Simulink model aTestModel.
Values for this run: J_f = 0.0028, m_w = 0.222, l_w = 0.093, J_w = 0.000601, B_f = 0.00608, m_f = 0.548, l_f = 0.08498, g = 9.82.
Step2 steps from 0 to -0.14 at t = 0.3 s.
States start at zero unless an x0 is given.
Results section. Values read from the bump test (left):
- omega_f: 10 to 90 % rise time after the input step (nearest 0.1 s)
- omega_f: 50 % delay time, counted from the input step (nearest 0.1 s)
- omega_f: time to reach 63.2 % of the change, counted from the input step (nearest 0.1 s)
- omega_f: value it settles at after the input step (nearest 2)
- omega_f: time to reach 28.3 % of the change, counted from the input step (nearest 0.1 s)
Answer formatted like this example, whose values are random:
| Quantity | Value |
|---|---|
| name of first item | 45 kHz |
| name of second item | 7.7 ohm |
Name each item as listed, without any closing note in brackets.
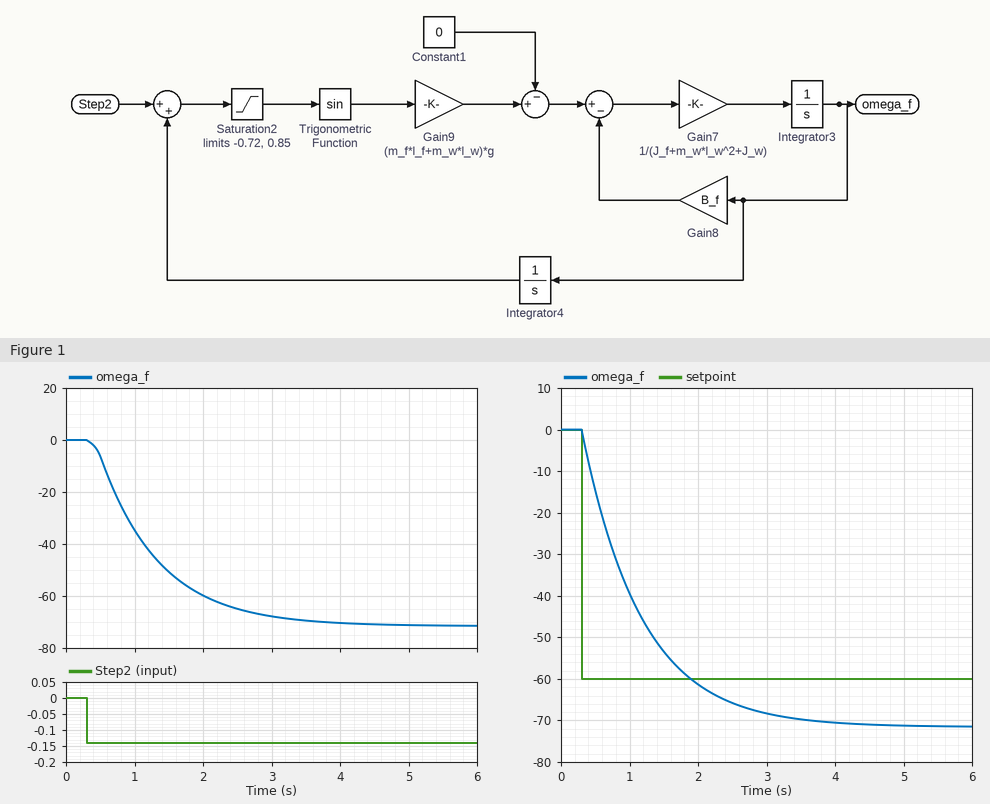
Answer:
| Quantity | Value |
|---|---|
| omega_f: 10 to 90 % rise time after the input step | 1.9 s |
| omega_f: 50 % delay time, counted from the input step | 0.7 s |
| omega_f: time to reach 63.2 % of the change, counted from the input step | 1.0 s |
| omega_f: value it settles at after the input step | -72 |
| omega_f: time to reach 28.3 % of the change, counted from the input step | 0.4 s |
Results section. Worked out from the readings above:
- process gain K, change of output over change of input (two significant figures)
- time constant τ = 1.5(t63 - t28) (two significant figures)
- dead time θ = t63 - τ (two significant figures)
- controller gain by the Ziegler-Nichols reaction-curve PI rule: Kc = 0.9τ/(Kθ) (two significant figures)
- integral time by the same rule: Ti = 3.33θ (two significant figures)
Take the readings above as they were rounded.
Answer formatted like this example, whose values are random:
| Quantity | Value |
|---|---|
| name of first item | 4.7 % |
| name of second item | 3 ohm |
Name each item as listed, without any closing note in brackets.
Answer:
| Quantity | Value |
|---|---|
| process gain K, change of output over change of input | 510 |
| time constant τ = 1.5(t63 - t28) | 0.90 s |
| dead time θ = t63 - τ | 0.10 s |
| controller gain by the Ziegler-Nichols reaction-curve PI rule: Kc = 0.9τ/(Kθ) | 0.016 |
| integral time by the same rule: Ti = 3.33θ | 0.33 s |
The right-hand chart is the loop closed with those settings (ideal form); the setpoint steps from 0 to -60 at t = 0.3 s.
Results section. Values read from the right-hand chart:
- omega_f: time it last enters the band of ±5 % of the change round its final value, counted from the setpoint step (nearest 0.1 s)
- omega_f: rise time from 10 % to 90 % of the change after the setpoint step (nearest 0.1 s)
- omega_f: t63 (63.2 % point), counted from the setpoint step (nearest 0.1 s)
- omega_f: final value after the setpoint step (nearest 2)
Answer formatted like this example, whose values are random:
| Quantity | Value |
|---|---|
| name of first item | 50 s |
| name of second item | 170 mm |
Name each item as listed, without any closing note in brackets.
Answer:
| Quantity | Value |
|---|---|
| omega_f: time it last enters the band of ±5 % of the change round its final value, counted from the setpoint step | 2.6 s |
| omega_f: rise time from 10 % to 90 % of the change after the setpoint step | 1.9 s |
| omega_f: t63 (63.2 % point), counted from the setpoint step | 0.9 s |
| omega_f: final value after the setpoint step | -72 |
